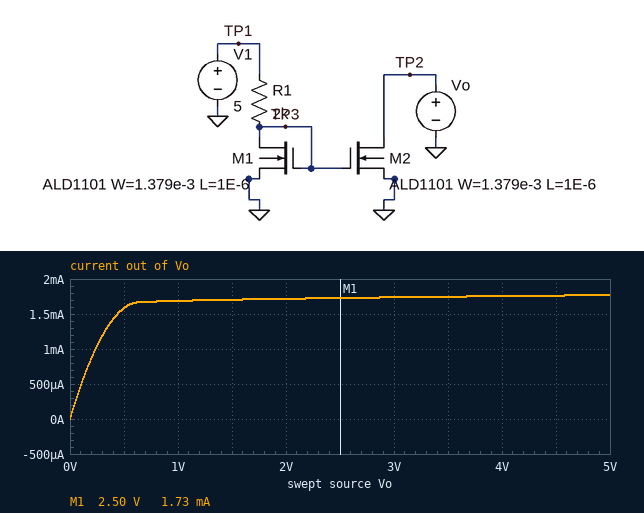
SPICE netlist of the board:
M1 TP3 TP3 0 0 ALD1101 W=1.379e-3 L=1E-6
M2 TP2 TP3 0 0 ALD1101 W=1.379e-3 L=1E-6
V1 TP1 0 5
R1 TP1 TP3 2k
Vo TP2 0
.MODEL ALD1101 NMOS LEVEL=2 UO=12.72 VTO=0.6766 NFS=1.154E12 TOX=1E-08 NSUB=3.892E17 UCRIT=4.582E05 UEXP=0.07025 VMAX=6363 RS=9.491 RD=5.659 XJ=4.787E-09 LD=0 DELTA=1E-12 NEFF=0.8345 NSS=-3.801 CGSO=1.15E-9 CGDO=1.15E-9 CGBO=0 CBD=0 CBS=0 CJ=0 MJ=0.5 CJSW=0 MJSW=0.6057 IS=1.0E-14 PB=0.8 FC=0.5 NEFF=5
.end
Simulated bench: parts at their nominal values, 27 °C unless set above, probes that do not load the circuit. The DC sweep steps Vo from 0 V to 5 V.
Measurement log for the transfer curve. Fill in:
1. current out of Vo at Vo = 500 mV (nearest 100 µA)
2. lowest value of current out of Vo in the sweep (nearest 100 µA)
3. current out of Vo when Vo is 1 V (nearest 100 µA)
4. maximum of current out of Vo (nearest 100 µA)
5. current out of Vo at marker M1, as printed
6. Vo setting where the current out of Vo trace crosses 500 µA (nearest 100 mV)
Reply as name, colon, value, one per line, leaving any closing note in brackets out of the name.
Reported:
current out of Vo at Vo = 500 mV: 1.6 mA
lowest value of current out of Vo in the sweep: 0 A
current out of Vo when Vo is 1 V: 1.7 mA
maximum of current out of Vo: 1.8 mA
current out of Vo at marker M1, as printed: 1.73 mA
Vo setting where the current out of Vo trace crosses 500 µA: 100 mV
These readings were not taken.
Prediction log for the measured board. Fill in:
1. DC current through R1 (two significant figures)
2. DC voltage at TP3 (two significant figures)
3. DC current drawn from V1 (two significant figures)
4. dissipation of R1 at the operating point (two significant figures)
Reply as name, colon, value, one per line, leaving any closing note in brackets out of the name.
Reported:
DC current through R1: 1.7 mA
DC voltage at TP3: 1.6 V
DC current drawn from V1: 1.7 mA
dissipation of R1 at the operating point: 5.8 mW
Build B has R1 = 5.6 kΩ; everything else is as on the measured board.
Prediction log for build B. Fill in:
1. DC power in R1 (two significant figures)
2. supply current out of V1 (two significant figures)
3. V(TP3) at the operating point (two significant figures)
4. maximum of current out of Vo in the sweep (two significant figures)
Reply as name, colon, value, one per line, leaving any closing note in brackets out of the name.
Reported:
DC power in R1: 2.5 mW
supply current out of V1: 670 µA
V(TP3) at the operating point: 1.2 V
maximum of current out of Vo in the sweep: 700 µA
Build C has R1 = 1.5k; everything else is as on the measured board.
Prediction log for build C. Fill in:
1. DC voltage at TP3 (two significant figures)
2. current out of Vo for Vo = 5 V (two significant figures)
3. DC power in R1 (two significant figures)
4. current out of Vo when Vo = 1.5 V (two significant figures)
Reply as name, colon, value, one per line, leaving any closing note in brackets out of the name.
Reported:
DC voltage at TP3: 1.7 V
current out of Vo for Vo = 5 V: 2.3 mA
DC power in R1: 7.2 mW
current out of Vo when Vo = 1.5 V: 2.2 mA
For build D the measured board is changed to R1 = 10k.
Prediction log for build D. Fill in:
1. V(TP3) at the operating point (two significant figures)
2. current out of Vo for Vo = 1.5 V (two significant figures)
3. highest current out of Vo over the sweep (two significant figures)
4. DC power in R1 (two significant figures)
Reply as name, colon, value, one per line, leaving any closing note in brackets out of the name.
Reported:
V(TP3) at the operating point: 1.1 V
current out of Vo for Vo = 1.5 V: 390 µA
highest current out of Vo over the sweep: 410 µA
DC power in R1: 1.5 mW
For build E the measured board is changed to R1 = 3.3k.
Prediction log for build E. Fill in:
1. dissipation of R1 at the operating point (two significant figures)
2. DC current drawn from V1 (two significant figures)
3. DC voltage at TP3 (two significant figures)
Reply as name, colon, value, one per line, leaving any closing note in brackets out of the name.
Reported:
dissipation of R1 at the operating point: 3.9 mW
DC current drawn from V1: 1.1 mA
DC voltage at TP3: 1.4 V
